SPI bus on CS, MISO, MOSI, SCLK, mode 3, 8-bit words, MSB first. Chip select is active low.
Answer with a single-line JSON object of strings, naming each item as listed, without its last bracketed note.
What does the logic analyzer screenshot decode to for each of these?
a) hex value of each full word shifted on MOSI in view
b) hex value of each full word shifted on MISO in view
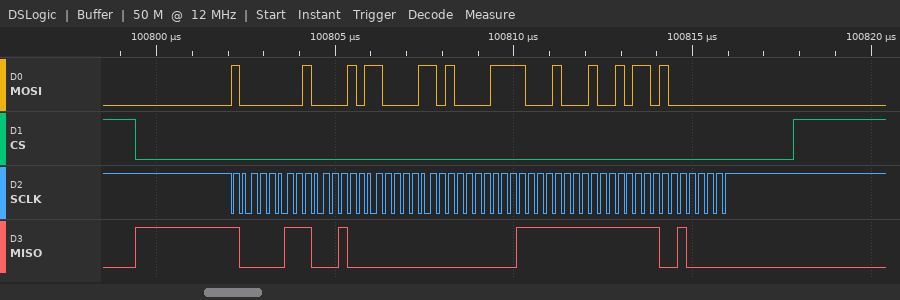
{"hex value of each full word shifted on MOSI in view": "80, 85, 86, 87, 88, 96, 80", "hex value of each full word shifted on MISO in view": "83, 88, 00, 00, FF, FF, 20"}
